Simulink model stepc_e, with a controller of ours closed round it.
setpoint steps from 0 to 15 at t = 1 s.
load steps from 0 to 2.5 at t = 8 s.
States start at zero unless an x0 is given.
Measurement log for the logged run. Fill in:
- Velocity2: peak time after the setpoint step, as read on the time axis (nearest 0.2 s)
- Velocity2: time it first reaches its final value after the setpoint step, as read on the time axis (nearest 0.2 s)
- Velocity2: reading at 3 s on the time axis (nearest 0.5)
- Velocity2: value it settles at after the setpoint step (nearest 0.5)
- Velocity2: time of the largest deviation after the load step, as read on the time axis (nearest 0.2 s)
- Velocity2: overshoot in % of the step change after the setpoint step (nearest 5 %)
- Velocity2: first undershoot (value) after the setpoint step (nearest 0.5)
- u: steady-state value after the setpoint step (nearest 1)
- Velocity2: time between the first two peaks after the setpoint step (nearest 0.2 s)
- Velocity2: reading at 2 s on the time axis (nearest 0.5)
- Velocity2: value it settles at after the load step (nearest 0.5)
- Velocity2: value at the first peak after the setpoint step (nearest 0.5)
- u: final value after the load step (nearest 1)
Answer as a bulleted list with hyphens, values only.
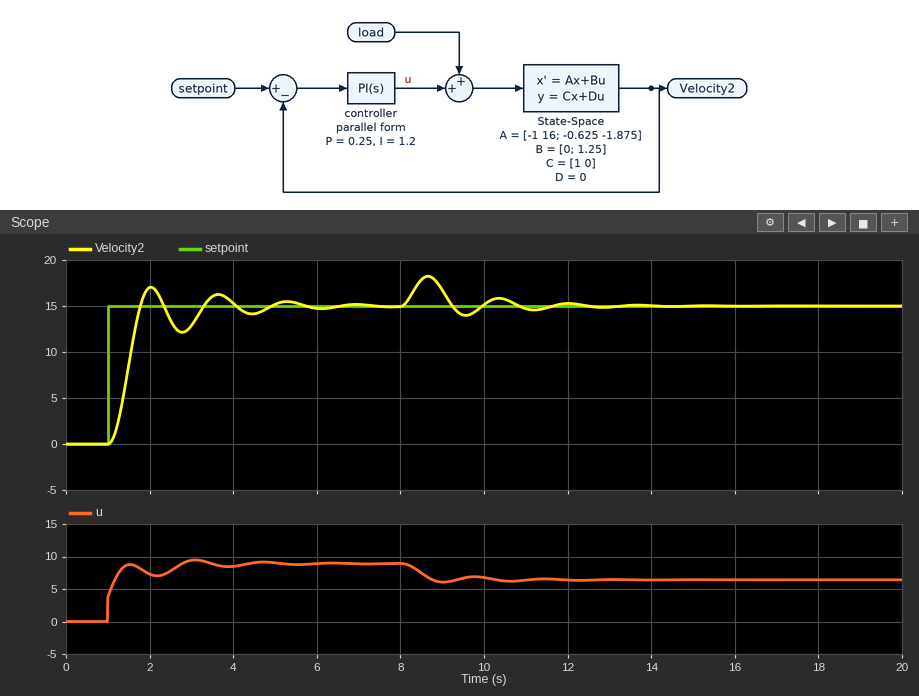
- 2.0 s
- 1.8 s
- 13.0
- 15.0
- 8.6 s
- 15 %
- 12.0
- 9
- 1.6 s
- 17.0
- 15.0
- 17.0
- 6
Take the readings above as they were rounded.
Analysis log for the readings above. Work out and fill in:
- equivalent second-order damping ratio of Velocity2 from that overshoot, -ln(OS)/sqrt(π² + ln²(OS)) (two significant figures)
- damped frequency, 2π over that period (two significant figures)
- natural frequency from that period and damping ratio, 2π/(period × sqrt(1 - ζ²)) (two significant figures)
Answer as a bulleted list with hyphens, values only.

- 0.52
- 3.9 rad/s
- 4.6 rad/s
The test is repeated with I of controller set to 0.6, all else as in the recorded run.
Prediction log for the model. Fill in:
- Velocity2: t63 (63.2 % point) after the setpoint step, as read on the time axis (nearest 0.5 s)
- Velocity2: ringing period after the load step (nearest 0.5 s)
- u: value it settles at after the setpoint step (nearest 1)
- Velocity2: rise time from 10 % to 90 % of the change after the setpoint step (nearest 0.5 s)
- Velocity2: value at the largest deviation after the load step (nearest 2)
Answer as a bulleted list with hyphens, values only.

- 1.5 s
- 1.5 s
- 9
- 2.0 s
- 18
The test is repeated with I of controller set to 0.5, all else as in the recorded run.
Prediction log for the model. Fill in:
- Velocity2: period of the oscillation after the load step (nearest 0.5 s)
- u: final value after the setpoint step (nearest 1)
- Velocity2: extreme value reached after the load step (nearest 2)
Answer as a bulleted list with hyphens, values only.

- 1.5 s
- 9
- 18
